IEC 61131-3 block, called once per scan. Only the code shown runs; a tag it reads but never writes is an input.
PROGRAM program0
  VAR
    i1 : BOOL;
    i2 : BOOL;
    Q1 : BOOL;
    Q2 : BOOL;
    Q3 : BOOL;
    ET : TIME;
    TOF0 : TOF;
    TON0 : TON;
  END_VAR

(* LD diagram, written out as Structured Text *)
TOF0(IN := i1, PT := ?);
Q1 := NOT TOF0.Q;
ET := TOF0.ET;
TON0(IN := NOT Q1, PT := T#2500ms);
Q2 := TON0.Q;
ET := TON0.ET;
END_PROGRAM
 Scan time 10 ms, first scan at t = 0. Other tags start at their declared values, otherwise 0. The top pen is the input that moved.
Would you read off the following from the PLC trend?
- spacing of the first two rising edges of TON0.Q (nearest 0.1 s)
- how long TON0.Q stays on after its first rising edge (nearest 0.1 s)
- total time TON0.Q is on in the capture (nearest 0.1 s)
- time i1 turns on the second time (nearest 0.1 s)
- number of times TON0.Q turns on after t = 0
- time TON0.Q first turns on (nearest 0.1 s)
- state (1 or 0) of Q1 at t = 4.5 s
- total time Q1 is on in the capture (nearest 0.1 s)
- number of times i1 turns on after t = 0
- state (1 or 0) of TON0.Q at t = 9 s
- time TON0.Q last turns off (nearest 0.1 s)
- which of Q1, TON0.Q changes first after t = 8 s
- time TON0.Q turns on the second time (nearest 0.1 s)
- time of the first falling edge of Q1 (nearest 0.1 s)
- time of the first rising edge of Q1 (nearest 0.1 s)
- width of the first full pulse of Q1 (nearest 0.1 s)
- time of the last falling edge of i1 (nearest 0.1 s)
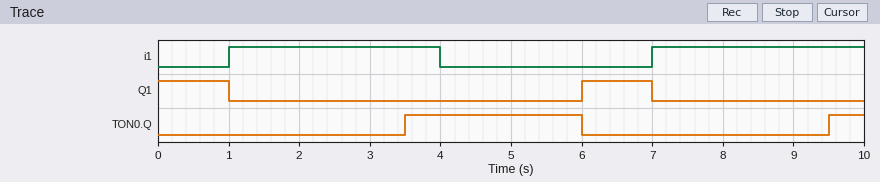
6.0 s
2.5 s
3.0 s
7.0 s
2
3.5 s
0
2.0 s
2
0
6.0 s
TON0.Q
9.5 s
1.0 s
6.0 s
1.0 s
4.0 s
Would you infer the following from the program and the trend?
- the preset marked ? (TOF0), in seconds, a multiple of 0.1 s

2.0 s
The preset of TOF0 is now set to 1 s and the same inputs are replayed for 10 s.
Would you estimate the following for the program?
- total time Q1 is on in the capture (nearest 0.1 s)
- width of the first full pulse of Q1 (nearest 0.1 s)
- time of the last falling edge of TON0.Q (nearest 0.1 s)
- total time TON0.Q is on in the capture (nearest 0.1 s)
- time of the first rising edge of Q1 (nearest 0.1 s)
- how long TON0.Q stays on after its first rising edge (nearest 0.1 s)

3.0 s
2.0 s
5.0 s
2.0 s
5.0 s
1.5 s
